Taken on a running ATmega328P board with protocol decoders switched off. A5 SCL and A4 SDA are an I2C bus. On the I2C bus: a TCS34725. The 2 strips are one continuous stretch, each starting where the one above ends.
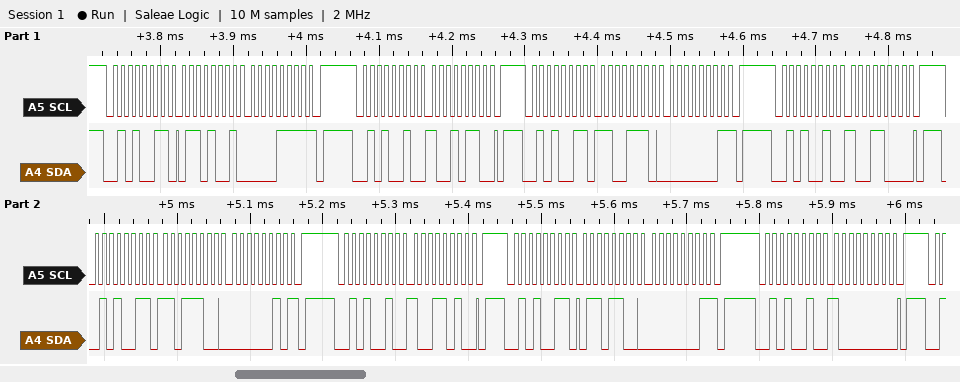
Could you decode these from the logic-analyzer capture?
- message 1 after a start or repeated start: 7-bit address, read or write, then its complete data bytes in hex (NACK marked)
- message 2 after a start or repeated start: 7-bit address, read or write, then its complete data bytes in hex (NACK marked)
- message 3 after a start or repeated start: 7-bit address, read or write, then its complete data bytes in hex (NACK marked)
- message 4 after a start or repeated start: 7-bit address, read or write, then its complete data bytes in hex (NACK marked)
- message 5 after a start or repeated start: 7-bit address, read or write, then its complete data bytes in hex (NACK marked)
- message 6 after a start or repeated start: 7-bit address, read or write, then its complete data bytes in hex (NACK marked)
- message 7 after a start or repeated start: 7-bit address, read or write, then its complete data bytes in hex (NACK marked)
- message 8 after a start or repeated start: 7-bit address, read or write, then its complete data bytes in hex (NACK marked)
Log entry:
0x29 read: 69 0F NACK
0x29 write: 96
0x29 read: CE 01 NACK
0x29 write: 98
0x29 read: DC 02 NACK
0x29 write: 9A
0x29 read: 6C 01 NACK
0x29 write: 80
